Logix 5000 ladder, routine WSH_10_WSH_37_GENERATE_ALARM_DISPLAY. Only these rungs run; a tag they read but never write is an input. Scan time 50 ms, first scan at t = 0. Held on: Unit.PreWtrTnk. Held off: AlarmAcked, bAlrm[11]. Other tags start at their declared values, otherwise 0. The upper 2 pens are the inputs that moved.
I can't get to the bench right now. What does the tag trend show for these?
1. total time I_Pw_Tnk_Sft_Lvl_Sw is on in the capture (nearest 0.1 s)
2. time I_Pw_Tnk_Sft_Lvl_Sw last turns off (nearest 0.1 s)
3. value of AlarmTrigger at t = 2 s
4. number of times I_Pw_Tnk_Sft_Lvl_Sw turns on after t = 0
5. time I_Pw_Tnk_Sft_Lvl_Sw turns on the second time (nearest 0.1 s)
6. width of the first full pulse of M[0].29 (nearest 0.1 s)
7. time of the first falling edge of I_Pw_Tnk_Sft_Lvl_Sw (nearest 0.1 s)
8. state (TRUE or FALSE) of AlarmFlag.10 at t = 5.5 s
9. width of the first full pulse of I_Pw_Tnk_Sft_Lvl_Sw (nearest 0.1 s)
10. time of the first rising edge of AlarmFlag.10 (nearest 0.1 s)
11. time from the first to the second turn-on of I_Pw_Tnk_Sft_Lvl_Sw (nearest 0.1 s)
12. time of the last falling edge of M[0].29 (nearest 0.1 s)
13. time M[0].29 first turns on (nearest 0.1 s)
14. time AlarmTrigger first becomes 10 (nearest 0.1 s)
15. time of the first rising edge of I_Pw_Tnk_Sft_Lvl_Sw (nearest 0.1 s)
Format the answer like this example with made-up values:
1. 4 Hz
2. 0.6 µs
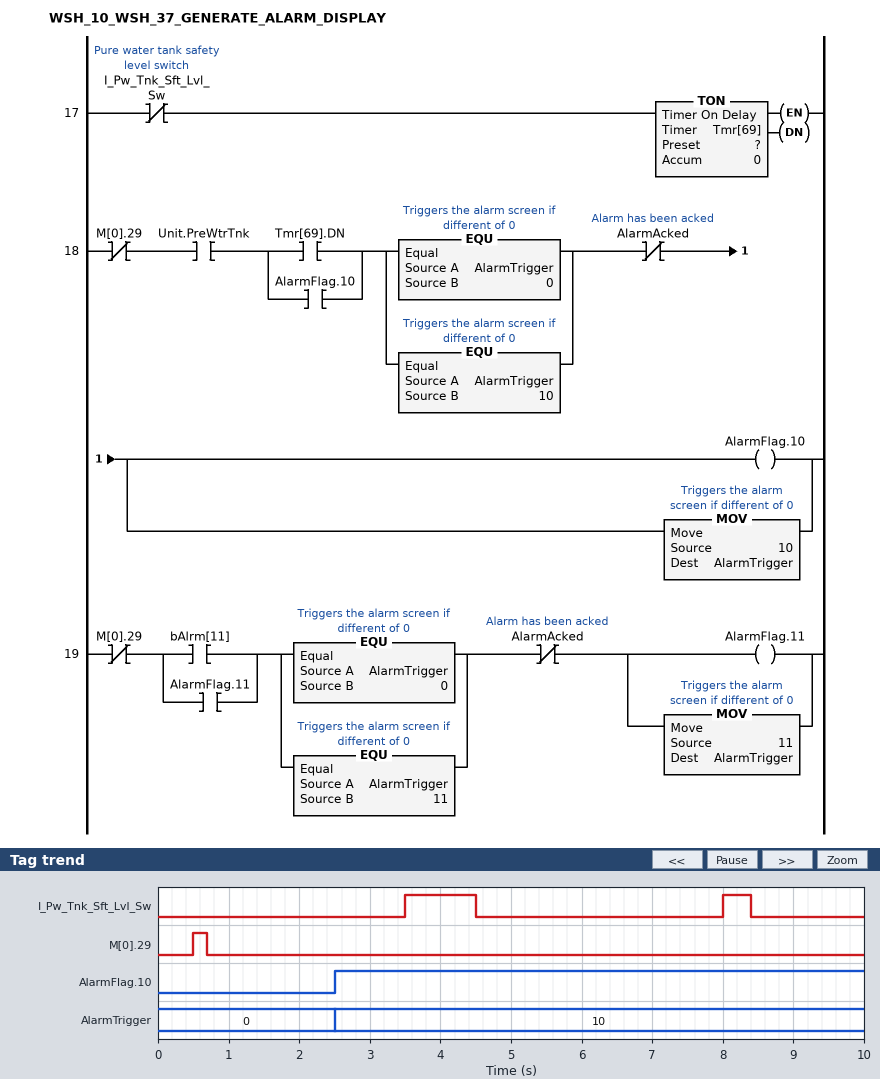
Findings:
1. 1.4 s
2. 8.4 s
3. 0
4. 2
5. 8.0 s
6. 0.2 s
7. 4.5 s
8. TRUE
9. 1.0 s
10. 2.5 s
11. 4.5 s
12. 0.7 s
13. 0.5 s
14. 2.5 s
15. 3.5 s
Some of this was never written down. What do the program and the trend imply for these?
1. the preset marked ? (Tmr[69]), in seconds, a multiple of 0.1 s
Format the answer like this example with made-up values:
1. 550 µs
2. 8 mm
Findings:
1. 2.5 s
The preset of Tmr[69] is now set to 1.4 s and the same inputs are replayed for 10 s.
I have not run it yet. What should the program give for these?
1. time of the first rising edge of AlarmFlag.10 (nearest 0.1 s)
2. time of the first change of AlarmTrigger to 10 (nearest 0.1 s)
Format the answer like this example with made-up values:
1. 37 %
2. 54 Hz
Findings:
1. 1.4 s
2. 1.4 s
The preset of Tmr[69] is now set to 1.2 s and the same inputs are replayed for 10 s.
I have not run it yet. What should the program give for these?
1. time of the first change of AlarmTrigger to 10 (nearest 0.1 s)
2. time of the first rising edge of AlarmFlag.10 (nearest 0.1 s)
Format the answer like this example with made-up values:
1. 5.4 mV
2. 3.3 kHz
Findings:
1. 1.2 s
2. 1.2 s
